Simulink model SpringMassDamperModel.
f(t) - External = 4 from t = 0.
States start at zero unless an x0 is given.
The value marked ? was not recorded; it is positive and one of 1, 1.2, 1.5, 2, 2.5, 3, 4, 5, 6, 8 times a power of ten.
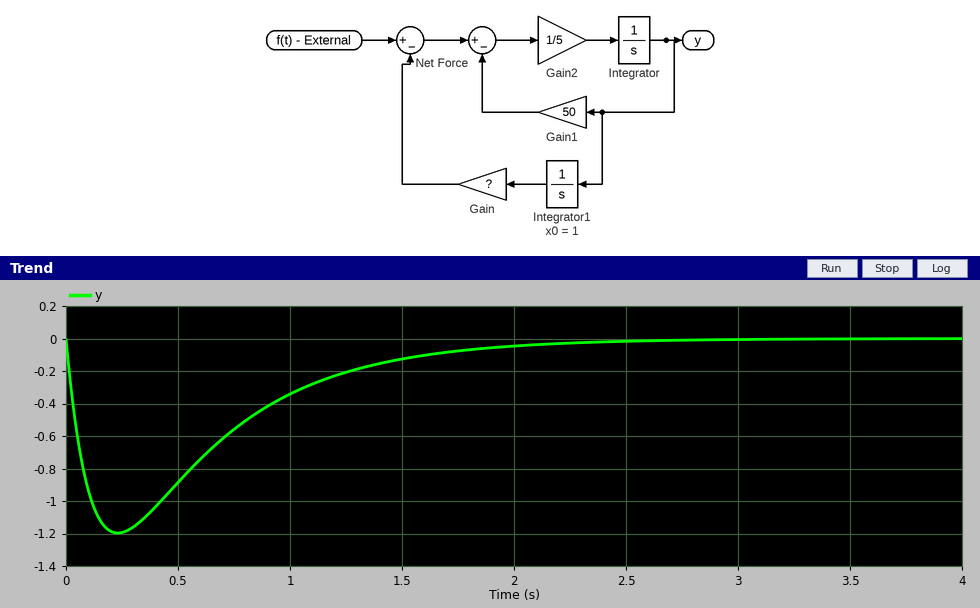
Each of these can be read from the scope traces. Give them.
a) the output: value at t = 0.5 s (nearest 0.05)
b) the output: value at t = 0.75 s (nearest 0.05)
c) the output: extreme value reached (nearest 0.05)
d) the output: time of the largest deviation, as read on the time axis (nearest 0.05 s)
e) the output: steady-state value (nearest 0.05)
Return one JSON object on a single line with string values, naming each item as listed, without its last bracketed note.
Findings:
{"the output: value at t = 0.5 s": "-0.90", "the output: value at t = 0.75 s": "-0.55", "the output: extreme value reached": "-1.20", "the output: time of the largest deviation, as read on the time axis": "0.25 s", "the output: steady-state value": "0.00"}
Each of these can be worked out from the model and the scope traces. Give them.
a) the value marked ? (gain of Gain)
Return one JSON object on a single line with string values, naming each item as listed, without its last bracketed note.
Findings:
{"the value marked ?": "80"}
